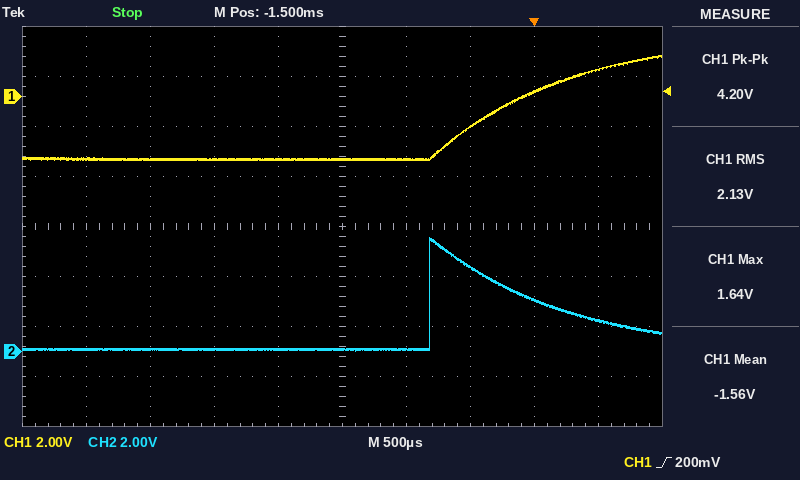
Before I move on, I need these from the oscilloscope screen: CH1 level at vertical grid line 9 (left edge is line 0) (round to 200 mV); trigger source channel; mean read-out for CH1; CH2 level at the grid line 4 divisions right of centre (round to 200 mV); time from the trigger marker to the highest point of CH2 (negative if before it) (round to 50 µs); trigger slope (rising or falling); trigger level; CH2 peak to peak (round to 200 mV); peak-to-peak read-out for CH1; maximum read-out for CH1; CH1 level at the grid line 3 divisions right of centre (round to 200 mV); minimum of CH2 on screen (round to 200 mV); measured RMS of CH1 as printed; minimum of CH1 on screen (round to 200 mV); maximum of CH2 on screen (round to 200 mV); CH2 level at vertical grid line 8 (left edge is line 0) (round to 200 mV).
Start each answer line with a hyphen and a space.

- 1.0 V
- CH1
- -1.56 V
- 1.2 V
- -800 µs
- rising
- 200 mV
- 4.6 V
- 4.20 V
- 1.64 V
- 200 mV
- 0.0 V
- 2.13 V
- -2.6 V
- 4.6 V
- 2.0 V
